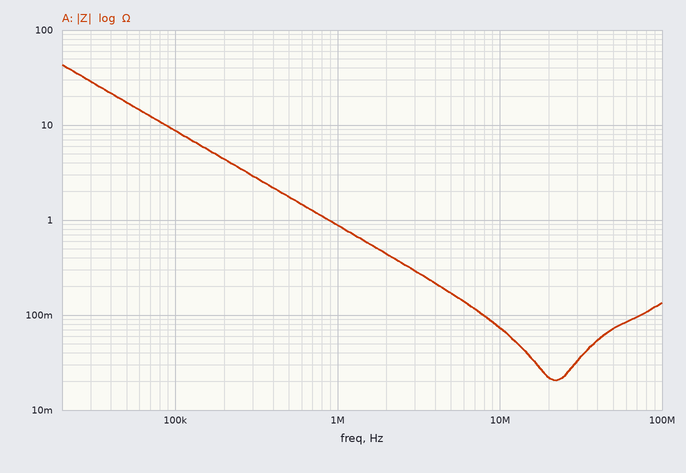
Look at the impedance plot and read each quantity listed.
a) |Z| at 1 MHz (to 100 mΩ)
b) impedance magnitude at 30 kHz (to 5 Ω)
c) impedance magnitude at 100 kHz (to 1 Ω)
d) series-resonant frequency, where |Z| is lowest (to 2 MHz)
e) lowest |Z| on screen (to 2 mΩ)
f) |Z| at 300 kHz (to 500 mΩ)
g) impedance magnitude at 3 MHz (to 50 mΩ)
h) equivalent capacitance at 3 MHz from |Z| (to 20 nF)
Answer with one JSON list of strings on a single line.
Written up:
["900 mΩ", "30 Ω", "9 Ω", "22 MHz", "20 mΩ", "3.0 Ω", "300 mΩ", "180 nF"]
